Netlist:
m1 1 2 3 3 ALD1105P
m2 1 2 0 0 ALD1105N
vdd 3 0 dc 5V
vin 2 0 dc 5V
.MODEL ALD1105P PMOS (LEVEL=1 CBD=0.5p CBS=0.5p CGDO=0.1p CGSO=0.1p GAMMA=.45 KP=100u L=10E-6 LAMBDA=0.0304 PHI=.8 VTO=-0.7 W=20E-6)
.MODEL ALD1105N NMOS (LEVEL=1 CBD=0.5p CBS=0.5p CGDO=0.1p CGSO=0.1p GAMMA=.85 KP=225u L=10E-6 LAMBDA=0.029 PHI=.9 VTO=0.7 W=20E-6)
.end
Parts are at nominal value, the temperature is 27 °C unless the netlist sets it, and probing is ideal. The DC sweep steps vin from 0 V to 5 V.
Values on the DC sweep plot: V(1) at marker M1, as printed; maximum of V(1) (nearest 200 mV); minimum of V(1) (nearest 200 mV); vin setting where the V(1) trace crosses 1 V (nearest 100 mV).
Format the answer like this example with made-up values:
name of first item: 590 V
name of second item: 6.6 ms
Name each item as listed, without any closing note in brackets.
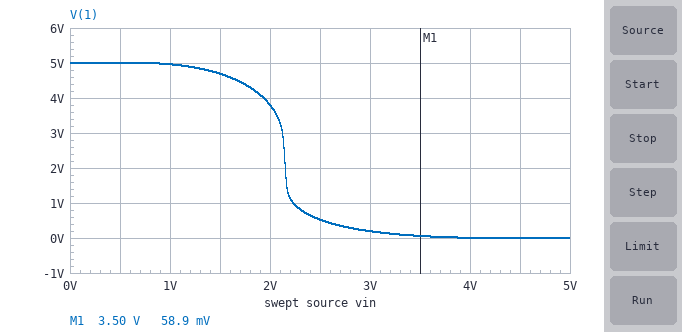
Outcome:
V(1) at marker M1, as printed: 58.9 mV
maximum of V(1): 5.0 V
minimum of V(1): 0 V
vin setting where the V(1) trace crosses 1 V: 2.2 V
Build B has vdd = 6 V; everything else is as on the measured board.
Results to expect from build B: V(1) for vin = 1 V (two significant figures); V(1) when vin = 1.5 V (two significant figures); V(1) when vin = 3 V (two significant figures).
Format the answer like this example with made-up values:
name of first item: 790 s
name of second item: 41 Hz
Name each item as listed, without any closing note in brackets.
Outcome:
V(1) for vin = 1 V: 6.0 V
V(1) when vin = 1.5 V: 5.8 V
V(1) when vin = 3 V: 680 mV
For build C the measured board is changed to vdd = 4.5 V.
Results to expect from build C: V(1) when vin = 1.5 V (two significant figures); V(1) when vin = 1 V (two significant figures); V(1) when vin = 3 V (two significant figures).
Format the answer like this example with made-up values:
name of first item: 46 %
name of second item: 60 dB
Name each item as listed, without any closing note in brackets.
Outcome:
V(1) when vin = 1.5 V: 4.1 V
V(1) when vin = 1 V: 4.5 V
V(1) when vin = 3 V: 71 mV
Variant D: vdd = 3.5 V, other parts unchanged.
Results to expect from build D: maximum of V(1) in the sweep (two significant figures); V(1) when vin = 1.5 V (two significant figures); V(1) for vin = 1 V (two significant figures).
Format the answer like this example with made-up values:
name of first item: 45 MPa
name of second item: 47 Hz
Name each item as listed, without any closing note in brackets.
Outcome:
maximum of V(1) in the sweep: 3.5 V
V(1) when vin = 1.5 V: 2.6 V
V(1) for vin = 1 V: 3.4 V
